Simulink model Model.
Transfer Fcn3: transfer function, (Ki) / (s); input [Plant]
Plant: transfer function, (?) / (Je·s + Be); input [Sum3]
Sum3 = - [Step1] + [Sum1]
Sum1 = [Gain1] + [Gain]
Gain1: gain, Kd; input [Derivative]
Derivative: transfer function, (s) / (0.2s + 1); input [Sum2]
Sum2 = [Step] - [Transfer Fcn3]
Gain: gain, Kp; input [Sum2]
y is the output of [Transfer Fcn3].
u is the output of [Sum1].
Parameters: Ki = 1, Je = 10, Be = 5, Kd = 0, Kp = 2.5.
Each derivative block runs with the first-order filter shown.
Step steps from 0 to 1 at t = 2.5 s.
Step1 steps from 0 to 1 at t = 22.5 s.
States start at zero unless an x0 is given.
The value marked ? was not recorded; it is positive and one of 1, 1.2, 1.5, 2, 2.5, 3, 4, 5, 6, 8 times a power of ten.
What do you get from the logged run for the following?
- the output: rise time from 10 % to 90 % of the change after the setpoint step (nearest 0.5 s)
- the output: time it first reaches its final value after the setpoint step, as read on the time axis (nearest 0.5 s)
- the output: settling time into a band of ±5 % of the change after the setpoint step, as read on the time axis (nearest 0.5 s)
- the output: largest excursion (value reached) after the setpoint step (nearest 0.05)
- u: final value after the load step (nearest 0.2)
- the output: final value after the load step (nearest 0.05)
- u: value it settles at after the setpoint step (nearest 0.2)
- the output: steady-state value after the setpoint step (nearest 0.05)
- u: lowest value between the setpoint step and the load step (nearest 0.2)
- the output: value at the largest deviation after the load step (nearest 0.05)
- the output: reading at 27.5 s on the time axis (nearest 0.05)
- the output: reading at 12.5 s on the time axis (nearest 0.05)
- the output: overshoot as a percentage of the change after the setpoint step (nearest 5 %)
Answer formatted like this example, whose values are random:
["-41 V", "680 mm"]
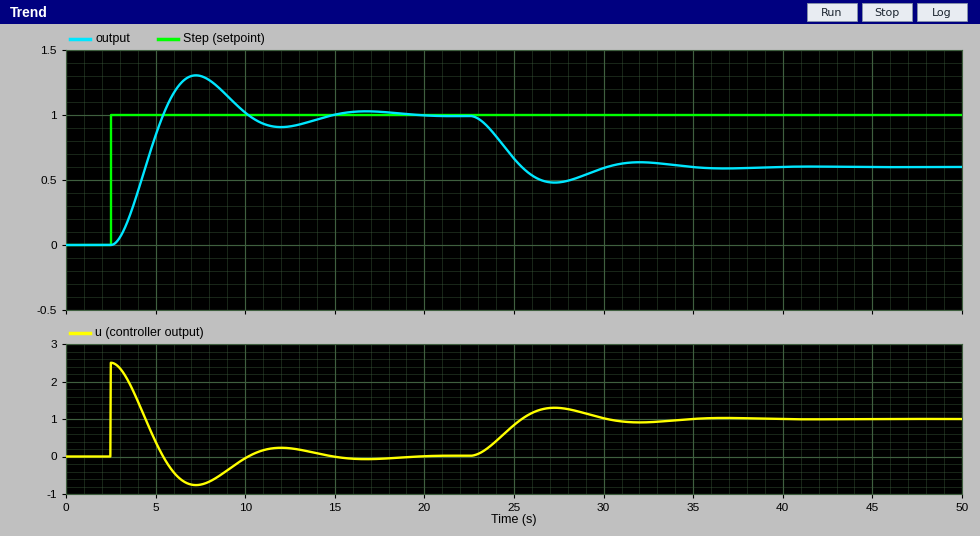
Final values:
["2.0 s", "5.5 s", "13.5 s", "1.30", "1.0", "0.60", "0.0", "1.00", "-0.8", "0.50", "0.50", "0.90", "30 %"]
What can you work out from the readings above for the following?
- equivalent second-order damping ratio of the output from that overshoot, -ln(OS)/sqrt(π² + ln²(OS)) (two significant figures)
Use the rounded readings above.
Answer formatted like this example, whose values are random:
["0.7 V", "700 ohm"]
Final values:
["0.36"]
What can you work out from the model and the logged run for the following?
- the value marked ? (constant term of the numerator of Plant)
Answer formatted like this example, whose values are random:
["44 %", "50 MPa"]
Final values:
["2"]
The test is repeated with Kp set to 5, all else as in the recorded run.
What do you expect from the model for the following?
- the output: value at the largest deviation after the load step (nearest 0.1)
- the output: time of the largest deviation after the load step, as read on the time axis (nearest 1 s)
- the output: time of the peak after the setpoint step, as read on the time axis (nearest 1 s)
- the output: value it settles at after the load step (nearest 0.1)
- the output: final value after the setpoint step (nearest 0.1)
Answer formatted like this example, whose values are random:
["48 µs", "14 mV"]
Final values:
["0.7", "26 s", "6 s", "0.8", "1.0"]
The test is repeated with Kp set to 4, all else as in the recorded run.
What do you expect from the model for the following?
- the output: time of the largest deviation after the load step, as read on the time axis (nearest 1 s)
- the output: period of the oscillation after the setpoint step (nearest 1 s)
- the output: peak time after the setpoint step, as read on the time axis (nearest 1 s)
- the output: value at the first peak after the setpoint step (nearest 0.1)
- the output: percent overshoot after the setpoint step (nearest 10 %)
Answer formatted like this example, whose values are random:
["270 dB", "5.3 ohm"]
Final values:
["26 s", "7 s", "6 s", "1.4", "40 %"]
